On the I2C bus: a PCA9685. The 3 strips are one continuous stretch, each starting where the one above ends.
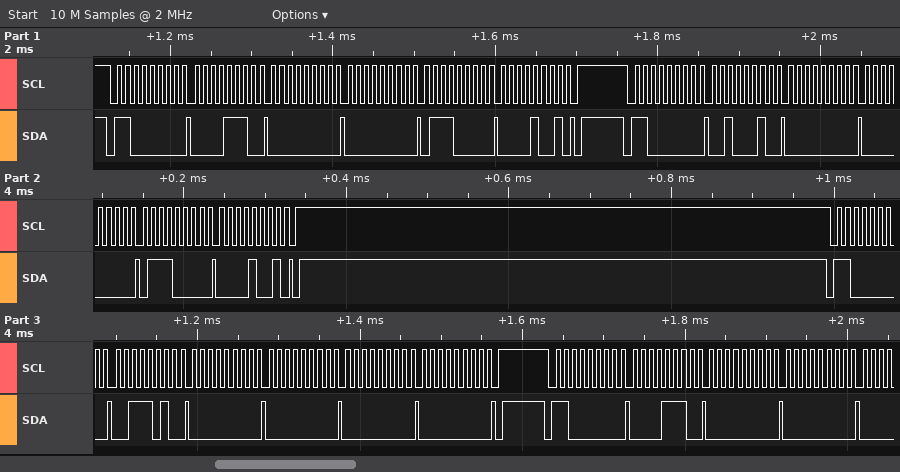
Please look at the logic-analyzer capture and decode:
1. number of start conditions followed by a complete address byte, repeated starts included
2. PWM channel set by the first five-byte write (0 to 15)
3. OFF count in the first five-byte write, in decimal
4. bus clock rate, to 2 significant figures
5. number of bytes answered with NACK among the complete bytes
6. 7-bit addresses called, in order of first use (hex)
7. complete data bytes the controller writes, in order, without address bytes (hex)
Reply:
4
2
2416
100 kHz
0
0x60
0E 00 00 70 09 22 00 00 70 09 3A 00 00 00 00 0E 00 00
